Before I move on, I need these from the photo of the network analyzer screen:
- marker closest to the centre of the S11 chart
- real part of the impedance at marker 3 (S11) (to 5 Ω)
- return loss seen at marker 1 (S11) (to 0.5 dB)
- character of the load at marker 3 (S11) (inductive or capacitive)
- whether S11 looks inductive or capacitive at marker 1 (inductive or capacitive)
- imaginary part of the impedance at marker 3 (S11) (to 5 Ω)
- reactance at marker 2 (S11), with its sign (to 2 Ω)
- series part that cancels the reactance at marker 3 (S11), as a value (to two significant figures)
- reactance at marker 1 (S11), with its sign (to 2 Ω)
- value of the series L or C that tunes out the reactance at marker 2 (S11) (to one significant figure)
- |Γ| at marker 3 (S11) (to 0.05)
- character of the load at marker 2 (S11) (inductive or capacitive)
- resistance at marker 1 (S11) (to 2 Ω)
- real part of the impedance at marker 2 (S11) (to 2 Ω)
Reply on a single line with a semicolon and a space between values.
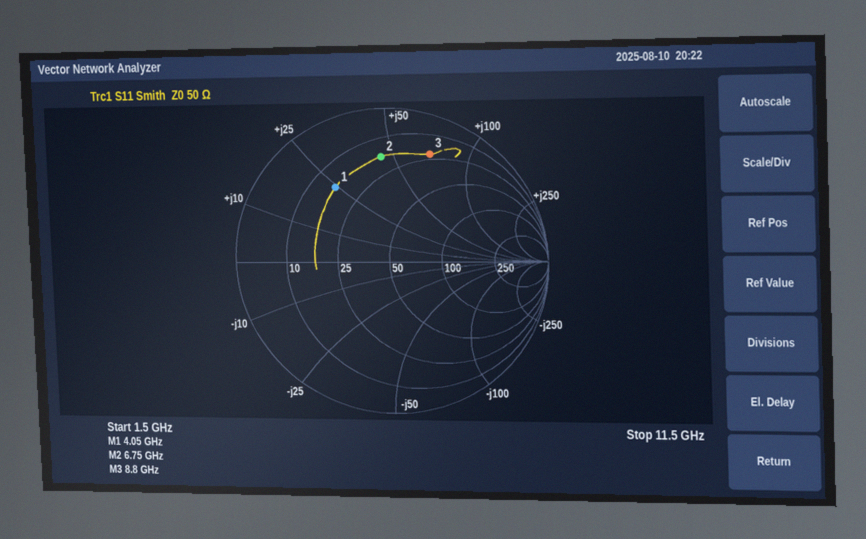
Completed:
marker 1; 20 Ω; 4.5 dB; inductive; inductive; +70 Ω; +44 Ω; 260 fF; +24 Ω; 500 fF; 0.75; inductive; 16 Ω; 18 Ω
